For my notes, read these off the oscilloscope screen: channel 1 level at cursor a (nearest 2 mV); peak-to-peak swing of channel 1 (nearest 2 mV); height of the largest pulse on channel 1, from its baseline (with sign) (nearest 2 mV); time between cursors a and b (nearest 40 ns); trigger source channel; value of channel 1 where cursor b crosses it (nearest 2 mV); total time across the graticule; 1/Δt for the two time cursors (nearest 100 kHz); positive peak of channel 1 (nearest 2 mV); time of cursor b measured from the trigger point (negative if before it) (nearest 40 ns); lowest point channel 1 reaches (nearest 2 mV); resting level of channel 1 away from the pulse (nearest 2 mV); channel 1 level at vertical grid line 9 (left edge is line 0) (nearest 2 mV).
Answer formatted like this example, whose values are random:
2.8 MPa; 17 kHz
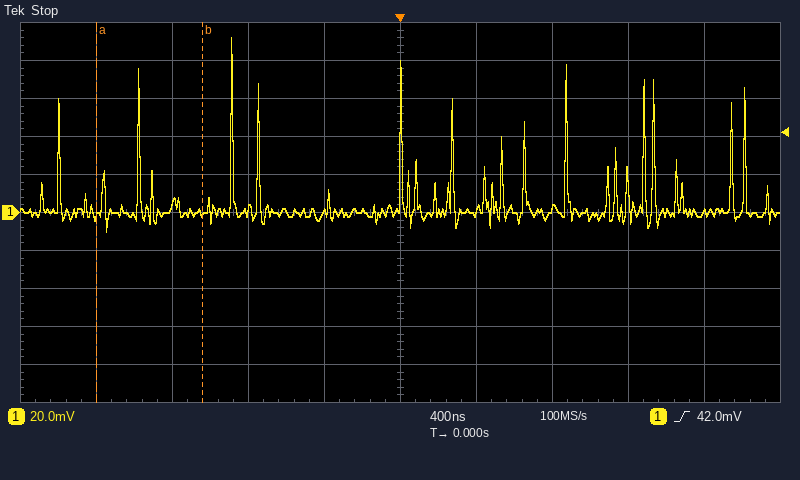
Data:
-2 mV; 102 mV; +92 mV; 560 ns; channel 1; 0 mV; 4 µs; 1.8 MHz; 92 mV; -1.04 µs; -10 mV; 0 mV; 0 mV
